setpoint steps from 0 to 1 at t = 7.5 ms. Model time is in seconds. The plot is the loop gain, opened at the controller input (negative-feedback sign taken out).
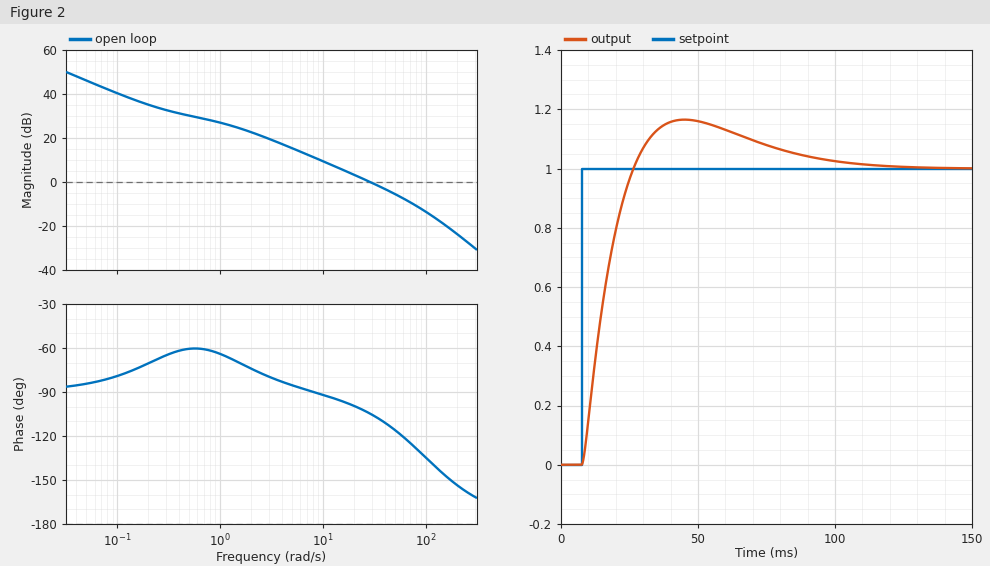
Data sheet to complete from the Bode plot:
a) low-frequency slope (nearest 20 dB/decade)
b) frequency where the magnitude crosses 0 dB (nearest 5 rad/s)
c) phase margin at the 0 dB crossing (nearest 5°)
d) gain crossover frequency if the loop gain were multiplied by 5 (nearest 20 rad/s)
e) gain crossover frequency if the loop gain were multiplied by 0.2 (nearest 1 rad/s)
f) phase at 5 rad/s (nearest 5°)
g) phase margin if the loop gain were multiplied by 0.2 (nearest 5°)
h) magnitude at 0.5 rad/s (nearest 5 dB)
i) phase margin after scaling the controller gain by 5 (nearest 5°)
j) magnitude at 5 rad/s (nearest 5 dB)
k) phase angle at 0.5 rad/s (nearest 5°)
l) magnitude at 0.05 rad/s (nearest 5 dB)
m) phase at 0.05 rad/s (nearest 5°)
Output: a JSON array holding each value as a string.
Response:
["-20 dB/decade", "30 rad/s", "75°", "100 rad/s", "6 rad/s", "-85°", "95°", "30 dB", "45°", "15 dB", "-60°", "45 dB", "-85°"]
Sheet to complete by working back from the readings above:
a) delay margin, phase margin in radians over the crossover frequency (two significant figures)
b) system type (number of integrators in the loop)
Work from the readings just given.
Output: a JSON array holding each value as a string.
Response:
["0.044 s", "1"]
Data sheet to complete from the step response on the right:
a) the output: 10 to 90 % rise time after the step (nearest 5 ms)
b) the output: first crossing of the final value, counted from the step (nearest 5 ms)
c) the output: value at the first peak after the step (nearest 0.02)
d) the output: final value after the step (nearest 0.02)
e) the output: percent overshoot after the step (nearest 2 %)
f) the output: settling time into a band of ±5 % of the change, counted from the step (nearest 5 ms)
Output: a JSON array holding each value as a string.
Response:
["15 ms", "20 ms", "1.16", "1.00", "16 %", "80 ms"]
